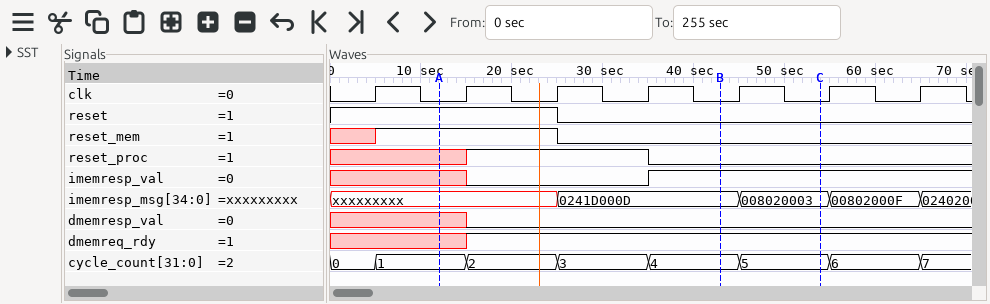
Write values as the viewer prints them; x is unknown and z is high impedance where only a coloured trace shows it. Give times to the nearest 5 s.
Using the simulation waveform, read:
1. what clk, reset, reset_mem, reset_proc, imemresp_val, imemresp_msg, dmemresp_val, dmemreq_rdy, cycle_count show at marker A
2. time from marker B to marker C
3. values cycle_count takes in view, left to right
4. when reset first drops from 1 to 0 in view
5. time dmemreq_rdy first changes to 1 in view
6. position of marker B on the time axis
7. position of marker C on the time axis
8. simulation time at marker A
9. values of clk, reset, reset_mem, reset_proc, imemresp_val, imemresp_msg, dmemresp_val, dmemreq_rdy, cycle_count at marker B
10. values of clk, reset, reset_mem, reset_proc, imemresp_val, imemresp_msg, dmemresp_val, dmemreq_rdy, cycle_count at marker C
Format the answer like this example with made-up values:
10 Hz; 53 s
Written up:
clk=0, reset=1, reset_mem=1, reset_proc=x, imemresp_val=x, imemresp_msg=xxxxxxxxx, dmemresp_val=x, dmemreq_rdy=x, cycle_count=1; 10 s; 0, 1, 2, 3, 4, 5, 6, 7; 25 s; 15 s; 45 s; 55 s; 10 s; clk=0, reset=0, reset_mem=0, reset_proc=0, imemresp_val=1, imemresp_msg=0241D000D, dmemresp_val=0, dmemreq_rdy=1, cycle_count=4; clk=0, reset=0, reset_mem=0, reset_proc=0, imemresp_val=1, imemresp_msg=008020003, dmemresp_val=0, dmemreq_rdy=1, cycle_count=5
